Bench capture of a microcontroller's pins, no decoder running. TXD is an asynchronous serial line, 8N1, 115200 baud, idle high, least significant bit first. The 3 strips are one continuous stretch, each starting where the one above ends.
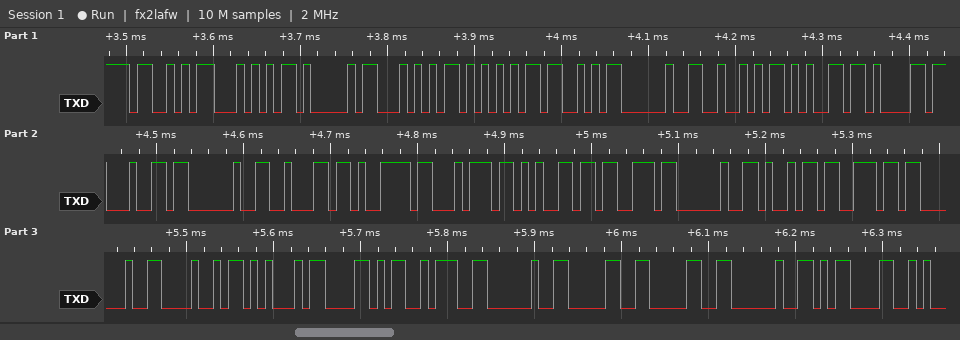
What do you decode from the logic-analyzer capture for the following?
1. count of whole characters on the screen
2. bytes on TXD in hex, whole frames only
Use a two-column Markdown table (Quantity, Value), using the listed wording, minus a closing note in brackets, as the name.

| Quantity | Value |
|---|---|
| count of whole characters on the screen | 30 |
| bytes on TXD in hex, whole frames only | 0x53 0x54 0x41 0x54 0x55 0x53 0x20 0x52 0x65 0x61 0x64 0x20 0x62 0x79 0x74 0x65 0x73 0x20 0x69 0x6E 0x20 0x48 0x45 0x58 0x3A 0x20 0x30 0x30 0x20 0x0D |
